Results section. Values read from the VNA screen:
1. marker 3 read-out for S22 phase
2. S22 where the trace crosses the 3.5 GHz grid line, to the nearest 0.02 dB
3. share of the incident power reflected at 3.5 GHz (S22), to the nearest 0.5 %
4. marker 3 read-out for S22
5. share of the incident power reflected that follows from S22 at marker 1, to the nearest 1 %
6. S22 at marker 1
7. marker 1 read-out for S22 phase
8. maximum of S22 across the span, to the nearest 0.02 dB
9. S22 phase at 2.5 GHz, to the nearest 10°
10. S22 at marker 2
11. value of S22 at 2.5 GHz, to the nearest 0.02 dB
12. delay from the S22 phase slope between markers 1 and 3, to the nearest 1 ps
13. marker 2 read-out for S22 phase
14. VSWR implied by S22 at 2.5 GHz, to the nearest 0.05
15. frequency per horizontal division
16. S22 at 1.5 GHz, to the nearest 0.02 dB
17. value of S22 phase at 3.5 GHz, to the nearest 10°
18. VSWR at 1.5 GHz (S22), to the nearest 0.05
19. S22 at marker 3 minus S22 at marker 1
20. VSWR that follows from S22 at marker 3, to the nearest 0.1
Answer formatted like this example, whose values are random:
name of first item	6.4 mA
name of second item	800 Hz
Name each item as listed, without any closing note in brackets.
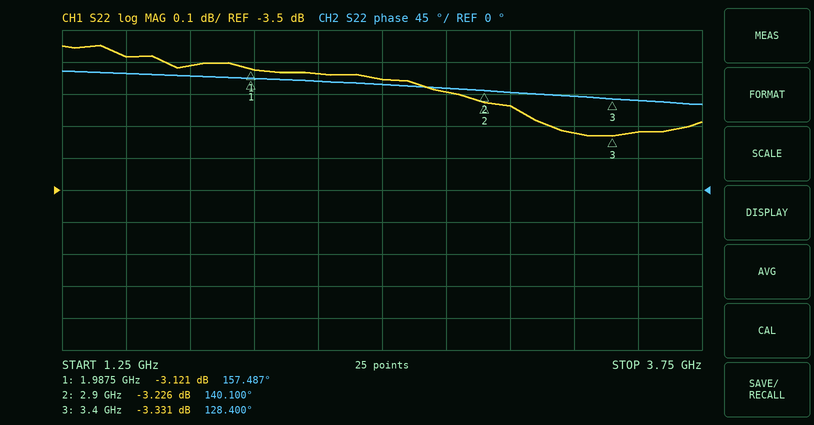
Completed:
marker 3 read-out for S22 phase	128.400°
S22 where the trace crosses the 3.5 GHz grid line, to the nearest 0.02 dB	-3.32 dB
share of the incident power reflected at 3.5 GHz (S22), to the nearest 0.5 %	46.5 %
marker 3 read-out for S22	-3.331 dB
share of the incident power reflected that follows from S22 at marker 1, to the nearest 1 %	49 %
S22 at marker 1	-3.121 dB
marker 1 read-out for S22 phase	157.487°
maximum of S22 across the span, to the nearest 0.02 dB	-3.04 dB
S22 phase at 2.5 GHz, to the nearest 10°	150°
S22 at marker 2	-3.226 dB
value of S22 at 2.5 GHz, to the nearest 0.02 dB	-3.16 dB
delay from the S22 phase slope between markers 1 and 3, to the nearest 1 ps	57 ps
marker 2 read-out for S22 phase	140.100°
VSWR implied by S22 at 2.5 GHz, to the nearest 0.05	5.55
frequency per horizontal division	250 MHz
S22 at 1.5 GHz, to the nearest 0.02 dB	-3.08 dB
value of S22 phase at 3.5 GHz, to the nearest 10°	130°
VSWR at 1.5 GHz (S22), to the nearest 0.05	5.70
S22 at marker 3 minus S22 at marker 1	-0.210 dB
VSWR that follows from S22 at marker 3, to the nearest 0.1	5.3
